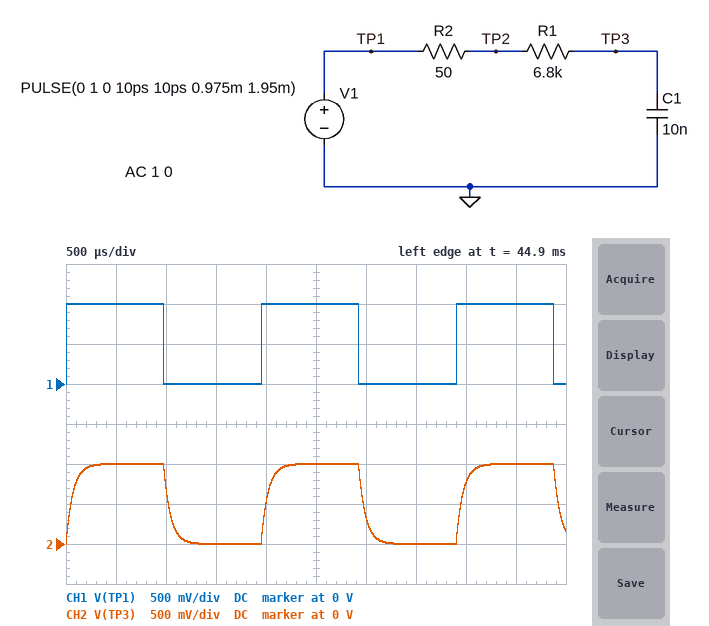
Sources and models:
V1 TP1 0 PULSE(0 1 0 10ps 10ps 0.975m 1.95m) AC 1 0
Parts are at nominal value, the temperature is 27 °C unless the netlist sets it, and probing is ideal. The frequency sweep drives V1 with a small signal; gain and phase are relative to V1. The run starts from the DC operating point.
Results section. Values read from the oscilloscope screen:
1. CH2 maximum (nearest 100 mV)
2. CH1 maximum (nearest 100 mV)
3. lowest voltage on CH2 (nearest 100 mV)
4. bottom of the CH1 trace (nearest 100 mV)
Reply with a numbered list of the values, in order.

1. 1.0 V
2. 1.0 V
3. 0 V
4. 0 V
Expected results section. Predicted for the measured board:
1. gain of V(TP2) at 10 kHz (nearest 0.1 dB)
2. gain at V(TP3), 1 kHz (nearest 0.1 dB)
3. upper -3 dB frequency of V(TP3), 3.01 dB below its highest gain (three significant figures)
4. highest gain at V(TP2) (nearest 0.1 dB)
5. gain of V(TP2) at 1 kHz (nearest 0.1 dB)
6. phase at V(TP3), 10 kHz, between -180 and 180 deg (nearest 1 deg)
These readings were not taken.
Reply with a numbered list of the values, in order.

1. -0.1 dB
2. -0.7 dB
3. 2.32 kHz
4. 0 dB
5. 0 dB
6. -77 deg
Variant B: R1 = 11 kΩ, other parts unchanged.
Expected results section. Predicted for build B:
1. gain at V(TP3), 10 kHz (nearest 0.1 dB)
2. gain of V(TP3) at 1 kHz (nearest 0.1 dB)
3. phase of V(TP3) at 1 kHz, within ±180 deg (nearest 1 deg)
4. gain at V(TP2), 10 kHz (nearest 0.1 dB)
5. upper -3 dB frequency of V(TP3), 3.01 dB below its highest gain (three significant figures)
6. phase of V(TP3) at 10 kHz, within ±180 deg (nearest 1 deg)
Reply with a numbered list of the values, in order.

1. -16.9 dB
2. -1.7 dB
3. -35 deg
4. 0 dB
5. 1.44 kHz
6. -82 deg
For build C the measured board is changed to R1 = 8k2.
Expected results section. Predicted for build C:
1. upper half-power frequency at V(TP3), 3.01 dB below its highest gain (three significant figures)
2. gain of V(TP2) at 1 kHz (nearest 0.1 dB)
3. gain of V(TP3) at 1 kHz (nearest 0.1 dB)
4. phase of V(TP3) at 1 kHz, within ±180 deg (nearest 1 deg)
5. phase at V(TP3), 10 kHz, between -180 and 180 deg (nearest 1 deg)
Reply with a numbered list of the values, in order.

1. 1.93 kHz
2. 0 dB
3. -1.0 dB
4. -27 deg
5. -79 deg
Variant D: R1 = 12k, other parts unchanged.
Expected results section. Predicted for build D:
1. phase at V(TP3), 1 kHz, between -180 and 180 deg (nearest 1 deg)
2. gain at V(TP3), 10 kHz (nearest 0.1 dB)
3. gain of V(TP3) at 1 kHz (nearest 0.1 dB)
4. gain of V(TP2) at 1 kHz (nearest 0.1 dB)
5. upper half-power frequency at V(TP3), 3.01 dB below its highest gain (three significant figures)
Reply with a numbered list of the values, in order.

1. -37 deg
2. -17.7 dB
3. -2.0 dB
4. 0 dB
5. 1.32 kHz
